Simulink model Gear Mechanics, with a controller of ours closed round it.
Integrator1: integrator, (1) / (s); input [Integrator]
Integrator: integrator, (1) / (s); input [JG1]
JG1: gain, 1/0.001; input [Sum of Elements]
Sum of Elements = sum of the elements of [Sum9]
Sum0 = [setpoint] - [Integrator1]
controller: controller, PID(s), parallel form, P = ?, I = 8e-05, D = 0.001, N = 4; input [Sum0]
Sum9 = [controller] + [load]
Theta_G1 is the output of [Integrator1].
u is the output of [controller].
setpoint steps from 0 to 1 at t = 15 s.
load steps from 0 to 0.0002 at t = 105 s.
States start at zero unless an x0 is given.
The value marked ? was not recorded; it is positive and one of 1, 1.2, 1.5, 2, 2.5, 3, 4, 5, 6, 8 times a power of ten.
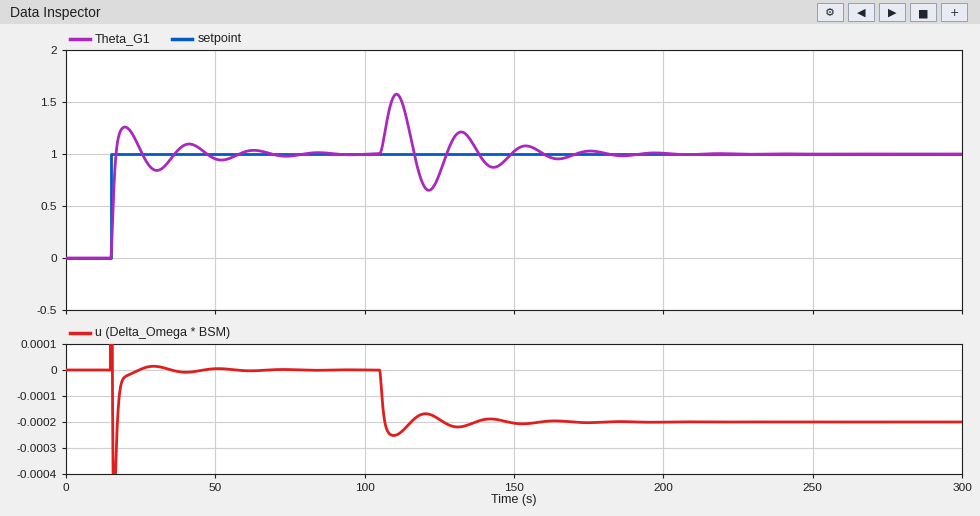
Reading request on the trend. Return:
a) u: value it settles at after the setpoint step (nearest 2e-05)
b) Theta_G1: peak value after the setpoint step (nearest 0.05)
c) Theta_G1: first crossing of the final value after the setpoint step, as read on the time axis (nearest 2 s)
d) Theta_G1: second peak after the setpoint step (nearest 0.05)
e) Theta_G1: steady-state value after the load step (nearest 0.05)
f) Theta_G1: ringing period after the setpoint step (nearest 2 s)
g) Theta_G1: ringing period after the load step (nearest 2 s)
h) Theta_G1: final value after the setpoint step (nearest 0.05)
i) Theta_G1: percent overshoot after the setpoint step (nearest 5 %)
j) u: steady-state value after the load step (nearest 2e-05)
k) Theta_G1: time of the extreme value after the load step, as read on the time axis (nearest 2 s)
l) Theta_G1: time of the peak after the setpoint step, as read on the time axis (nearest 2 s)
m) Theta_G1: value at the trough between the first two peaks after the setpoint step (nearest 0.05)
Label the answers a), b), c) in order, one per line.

a) 0.00000
b) 1.25
c) 16 s
d) 1.10
e) 1.00
f) 22 s
g) 22 s
h) 1.00
i) 25 %
j) -0.00020
k) 110 s
l) 20 s
m) 0.85
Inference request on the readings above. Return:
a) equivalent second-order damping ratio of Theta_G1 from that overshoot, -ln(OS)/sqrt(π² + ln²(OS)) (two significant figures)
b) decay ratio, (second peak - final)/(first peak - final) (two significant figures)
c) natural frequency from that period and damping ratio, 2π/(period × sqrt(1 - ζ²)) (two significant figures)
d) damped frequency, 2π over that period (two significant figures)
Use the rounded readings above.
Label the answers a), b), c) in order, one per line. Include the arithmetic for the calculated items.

a) ln(0.25) = -1.386; 1.386 / sqrt(9.870 + 1.922) = 0.40
b) (1.1 - 1) / (1.25 - 1) = 0.40
c) 2π / (22 × sqrt(1 - 0.4²)) = 0.31 rad/s
d) 2π / 22 = 0.29 rad/s
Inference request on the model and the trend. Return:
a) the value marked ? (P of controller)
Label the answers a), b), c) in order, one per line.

a) 0.00015
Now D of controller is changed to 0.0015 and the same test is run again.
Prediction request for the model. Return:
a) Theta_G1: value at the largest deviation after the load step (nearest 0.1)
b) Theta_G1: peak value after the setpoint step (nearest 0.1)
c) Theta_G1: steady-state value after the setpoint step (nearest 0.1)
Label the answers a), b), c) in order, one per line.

a) 1.5
b) 1.1
c) 1.0
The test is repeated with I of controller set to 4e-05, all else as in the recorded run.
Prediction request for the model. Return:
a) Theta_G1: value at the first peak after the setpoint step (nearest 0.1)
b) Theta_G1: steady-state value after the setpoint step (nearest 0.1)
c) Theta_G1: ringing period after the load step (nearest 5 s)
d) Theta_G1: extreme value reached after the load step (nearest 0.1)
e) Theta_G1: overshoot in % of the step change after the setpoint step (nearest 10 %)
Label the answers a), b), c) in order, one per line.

a) 1.2
b) 1.0
c) 30 s
d) 1.7
e) 20 %
